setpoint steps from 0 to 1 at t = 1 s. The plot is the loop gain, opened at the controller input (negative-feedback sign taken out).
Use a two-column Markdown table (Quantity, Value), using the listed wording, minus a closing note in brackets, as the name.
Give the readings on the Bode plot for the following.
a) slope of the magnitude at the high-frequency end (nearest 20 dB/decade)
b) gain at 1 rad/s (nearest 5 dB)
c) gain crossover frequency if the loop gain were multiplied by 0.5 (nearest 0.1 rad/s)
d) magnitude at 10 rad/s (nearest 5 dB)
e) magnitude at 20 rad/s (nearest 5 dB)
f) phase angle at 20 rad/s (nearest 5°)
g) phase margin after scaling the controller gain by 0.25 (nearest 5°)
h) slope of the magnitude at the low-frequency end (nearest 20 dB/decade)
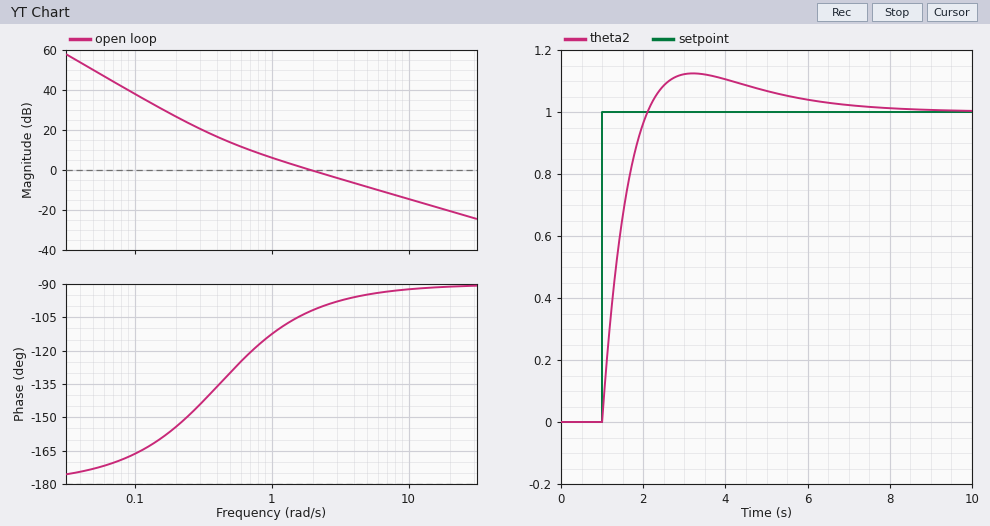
| Quantity | Value |
|---|---|
| slope of the magnitude at the high-frequency end | -20 dB/decade |
| gain at 1 rad/s | 5 dB |
| gain crossover frequency if the loop gain were multiplied by 0.5 | 1.0 rad/s |
| magnitude at 10 rad/s | -15 dB |
| magnitude at 20 rad/s | -20 dB |
| phase angle at 20 rad/s | -90° |
| phase margin after scaling the controller gain by 0.25 | 55° |
| slope of the magnitude at the low-frequency end | -40 dB/decade |
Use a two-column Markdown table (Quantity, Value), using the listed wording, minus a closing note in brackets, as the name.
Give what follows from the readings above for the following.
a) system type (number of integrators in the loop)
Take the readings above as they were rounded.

| Quantity | Value |
|---|---|
| system type | 2 |
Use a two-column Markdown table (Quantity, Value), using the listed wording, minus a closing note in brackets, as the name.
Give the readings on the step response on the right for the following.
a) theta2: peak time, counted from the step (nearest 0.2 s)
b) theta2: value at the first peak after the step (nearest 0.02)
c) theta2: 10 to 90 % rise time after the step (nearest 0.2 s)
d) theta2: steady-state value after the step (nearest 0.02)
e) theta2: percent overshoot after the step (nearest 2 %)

| Quantity | Value |
|---|---|
| theta2: peak time, counted from the step | 2.2 s |
| theta2: value at the first peak after the step | 1.12 |
| theta2: 10 to 90 % rise time after the step | 0.8 s |
| theta2: steady-state value after the step | 1.00 |
| theta2: percent overshoot after the step | 12 % |
